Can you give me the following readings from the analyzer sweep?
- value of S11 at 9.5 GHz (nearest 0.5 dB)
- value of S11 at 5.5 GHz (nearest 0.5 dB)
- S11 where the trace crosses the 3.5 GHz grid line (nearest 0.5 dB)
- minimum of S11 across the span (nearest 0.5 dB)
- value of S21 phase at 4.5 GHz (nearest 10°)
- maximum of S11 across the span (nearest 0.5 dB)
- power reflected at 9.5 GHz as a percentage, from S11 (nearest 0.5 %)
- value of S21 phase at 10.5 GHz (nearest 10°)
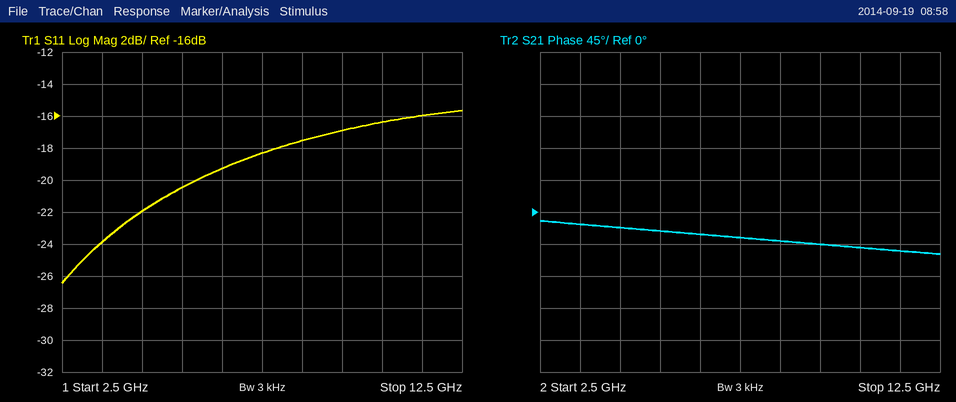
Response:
-17.0 dB
-20.5 dB
-24.0 dB
-26.5 dB
-20°
-15.5 dB
2.0 %
-50°
